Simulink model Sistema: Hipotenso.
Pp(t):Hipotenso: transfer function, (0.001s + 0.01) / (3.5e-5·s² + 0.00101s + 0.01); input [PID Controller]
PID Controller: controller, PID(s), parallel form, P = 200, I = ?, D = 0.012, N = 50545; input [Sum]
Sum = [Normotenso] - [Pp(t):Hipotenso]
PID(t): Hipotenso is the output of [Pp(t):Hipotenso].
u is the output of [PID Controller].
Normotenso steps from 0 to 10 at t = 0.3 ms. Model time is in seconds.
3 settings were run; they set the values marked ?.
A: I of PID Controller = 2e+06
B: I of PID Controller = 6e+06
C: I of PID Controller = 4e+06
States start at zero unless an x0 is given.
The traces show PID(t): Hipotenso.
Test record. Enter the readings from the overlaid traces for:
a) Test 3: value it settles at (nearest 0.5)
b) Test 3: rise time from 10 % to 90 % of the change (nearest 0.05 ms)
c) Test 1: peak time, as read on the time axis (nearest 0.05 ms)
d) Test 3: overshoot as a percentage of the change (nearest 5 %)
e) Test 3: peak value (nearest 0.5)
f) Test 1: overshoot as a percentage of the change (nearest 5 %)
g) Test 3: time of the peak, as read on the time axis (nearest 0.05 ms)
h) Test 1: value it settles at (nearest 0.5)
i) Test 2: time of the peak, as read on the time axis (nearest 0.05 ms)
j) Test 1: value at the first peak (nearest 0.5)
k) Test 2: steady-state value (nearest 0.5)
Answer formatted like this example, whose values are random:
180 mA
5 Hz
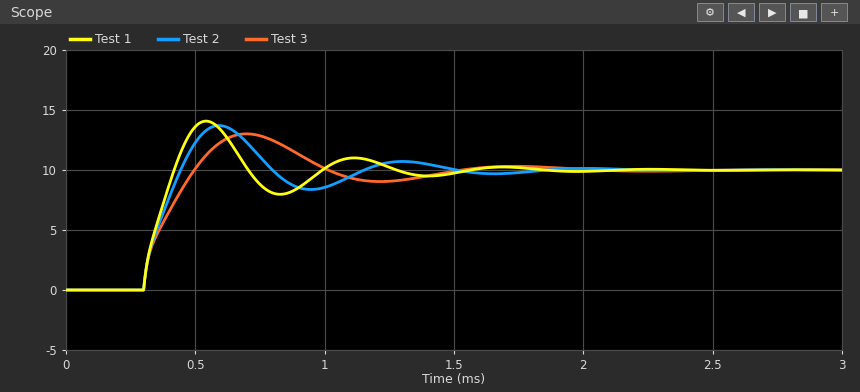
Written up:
10.0
0.15 ms
0.55 ms
30 %
13.0
40 %
0.70 ms
10.0
0.60 ms
14.0
10.0
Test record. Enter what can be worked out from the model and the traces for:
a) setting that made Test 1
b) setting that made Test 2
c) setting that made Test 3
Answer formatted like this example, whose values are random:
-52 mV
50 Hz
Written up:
B
C
A
